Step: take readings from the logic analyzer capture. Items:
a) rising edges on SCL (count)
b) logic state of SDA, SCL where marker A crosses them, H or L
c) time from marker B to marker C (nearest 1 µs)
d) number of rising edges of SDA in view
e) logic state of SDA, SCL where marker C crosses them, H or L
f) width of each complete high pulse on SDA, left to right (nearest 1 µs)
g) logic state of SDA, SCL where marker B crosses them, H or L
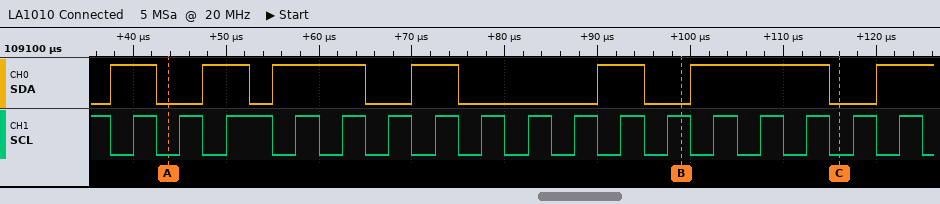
17
SDA=L, SCL=L
17 µs
7
SDA=L, SCL=L
5 µs, 5 µs, 10 µs, 5 µs, 5 µs, 15 µs
SDA=L, SCL=H
